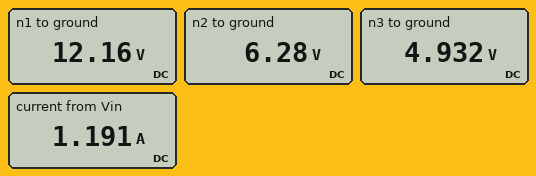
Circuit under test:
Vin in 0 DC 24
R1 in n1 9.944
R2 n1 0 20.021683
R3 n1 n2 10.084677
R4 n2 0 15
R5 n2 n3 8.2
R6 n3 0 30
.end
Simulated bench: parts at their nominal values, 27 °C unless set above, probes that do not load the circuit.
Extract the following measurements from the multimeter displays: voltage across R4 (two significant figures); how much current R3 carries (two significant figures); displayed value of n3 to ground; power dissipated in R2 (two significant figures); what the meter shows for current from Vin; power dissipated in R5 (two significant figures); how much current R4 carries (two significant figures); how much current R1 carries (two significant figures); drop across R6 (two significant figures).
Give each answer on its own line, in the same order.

6.3 V
580 mA
4.932 V
7.4 W
1.191 A
220 mW
420 mA
1.2 A
4.9 V
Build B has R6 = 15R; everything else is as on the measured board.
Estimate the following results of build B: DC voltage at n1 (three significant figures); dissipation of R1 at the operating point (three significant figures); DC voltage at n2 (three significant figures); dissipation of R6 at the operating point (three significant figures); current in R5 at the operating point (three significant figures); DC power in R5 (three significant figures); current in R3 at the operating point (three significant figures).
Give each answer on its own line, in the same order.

11.9 V
14.7 W
5.65 V
891 mW
244 mA
487 mW
621 mA
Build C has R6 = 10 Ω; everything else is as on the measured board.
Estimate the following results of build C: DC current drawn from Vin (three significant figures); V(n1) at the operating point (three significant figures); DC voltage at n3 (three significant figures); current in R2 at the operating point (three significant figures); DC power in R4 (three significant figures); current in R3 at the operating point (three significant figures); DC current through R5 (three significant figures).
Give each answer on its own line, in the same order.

1.23 A
11.8 V
2.90 V
588 mA
1.86 W
643 mA
290 mA
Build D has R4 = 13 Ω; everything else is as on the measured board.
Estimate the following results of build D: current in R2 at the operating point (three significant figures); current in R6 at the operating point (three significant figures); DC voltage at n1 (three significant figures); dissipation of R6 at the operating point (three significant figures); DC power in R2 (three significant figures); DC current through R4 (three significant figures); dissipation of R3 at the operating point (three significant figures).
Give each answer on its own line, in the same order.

600 mA
154 mA
12.0 V
712 mW
7.20 W
453 mA
3.71 W
